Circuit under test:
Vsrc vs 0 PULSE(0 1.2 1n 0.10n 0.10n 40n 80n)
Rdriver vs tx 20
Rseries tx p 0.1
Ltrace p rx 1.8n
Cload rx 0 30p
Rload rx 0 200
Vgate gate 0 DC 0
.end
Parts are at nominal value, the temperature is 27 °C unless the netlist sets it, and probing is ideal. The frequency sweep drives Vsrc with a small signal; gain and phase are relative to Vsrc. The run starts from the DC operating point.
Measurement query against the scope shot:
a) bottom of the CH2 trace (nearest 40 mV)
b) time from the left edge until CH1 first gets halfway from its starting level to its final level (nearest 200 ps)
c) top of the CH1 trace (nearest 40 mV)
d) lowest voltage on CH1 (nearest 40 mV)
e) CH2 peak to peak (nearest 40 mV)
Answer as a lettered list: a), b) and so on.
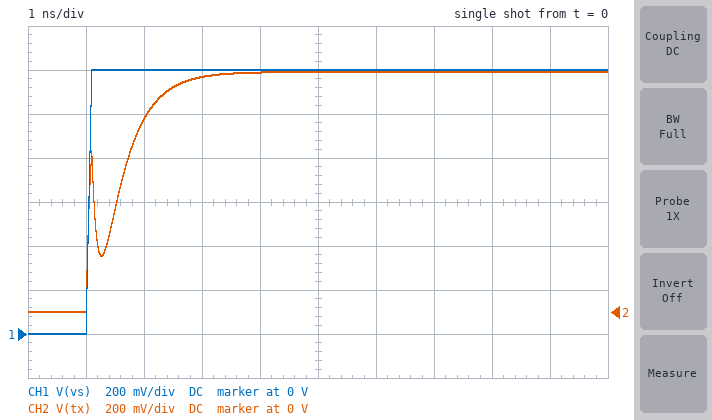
a) 0 V
b) 1.0 ns
c) 1.20 V
d) 0 V
e) 1.08 V
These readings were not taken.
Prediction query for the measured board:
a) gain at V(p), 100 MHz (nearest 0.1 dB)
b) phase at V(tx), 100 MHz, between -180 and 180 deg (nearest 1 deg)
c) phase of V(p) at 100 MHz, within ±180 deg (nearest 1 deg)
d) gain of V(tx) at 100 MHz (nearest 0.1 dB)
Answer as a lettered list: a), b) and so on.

a) -1.4 dB
b) -19 deg
c) -19 deg
d) -1.4 dB
